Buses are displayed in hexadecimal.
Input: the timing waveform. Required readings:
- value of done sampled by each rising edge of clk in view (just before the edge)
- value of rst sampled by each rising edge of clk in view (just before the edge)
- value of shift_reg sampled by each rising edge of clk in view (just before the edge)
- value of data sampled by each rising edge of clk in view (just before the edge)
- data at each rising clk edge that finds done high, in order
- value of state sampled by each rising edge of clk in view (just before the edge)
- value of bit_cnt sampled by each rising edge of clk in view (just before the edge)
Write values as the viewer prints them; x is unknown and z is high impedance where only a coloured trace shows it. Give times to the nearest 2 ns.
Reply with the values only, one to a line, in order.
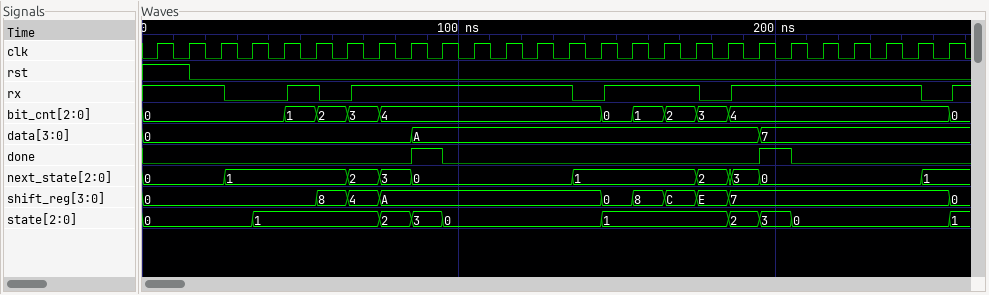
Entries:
0 0 0 0 0 0 0 0 0 1 0 0 0 0 0 0 0 0 0 0 1 0 0 0 0 0
1 1 0 0 0 0 0 0 0 0 0 0 0 0 0 0 0 0 0 0 0 0 0 0 0 0
0, 0, 0, 0, 0, 0, 8, 4, A, A, A, A, A, A, A, 0, 8, C, E, 7, 7, 7, 7, 7, 7, 7
0, 0, 0, 0, 0, 0, 0, 0, 0, A, A, A, A, A, A, A, A, A, A, A, 7, 7, 7, 7, 7, 7
A, 7
0, 0, 0, 0, 1, 1, 1, 1, 2, 3, 0, 0, 0, 0, 0, 1, 1, 1, 1, 2, 3, 0, 0, 0, 0, 0
0, 0, 0, 0, 0, 1, 2, 3, 4, 4, 4, 4, 4, 4, 4, 0, 1, 2, 3, 4, 4, 4, 4, 4, 4, 4
